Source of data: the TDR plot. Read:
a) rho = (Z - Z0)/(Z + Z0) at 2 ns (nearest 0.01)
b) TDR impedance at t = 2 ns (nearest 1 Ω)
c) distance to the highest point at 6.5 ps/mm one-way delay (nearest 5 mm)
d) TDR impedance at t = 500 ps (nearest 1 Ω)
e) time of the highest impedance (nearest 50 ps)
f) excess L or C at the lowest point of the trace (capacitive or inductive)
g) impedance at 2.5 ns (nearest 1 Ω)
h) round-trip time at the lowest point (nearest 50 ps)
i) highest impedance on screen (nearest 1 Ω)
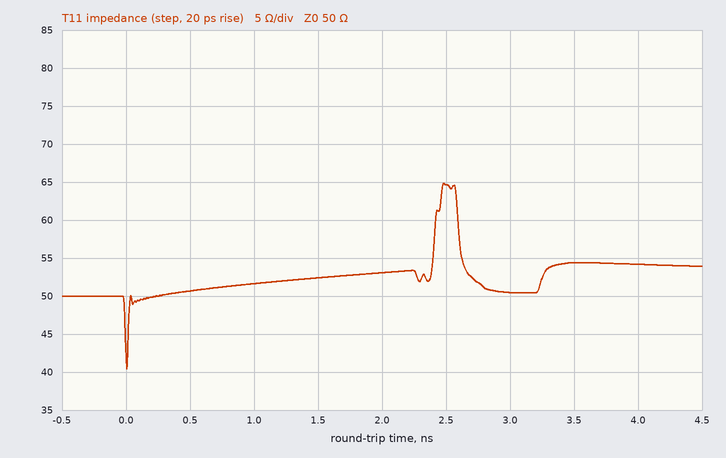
+0.03
53 Ω
190 mm
51 Ω
2.50 ns
capacitive
65 Ω
0 ps
65 Ω
